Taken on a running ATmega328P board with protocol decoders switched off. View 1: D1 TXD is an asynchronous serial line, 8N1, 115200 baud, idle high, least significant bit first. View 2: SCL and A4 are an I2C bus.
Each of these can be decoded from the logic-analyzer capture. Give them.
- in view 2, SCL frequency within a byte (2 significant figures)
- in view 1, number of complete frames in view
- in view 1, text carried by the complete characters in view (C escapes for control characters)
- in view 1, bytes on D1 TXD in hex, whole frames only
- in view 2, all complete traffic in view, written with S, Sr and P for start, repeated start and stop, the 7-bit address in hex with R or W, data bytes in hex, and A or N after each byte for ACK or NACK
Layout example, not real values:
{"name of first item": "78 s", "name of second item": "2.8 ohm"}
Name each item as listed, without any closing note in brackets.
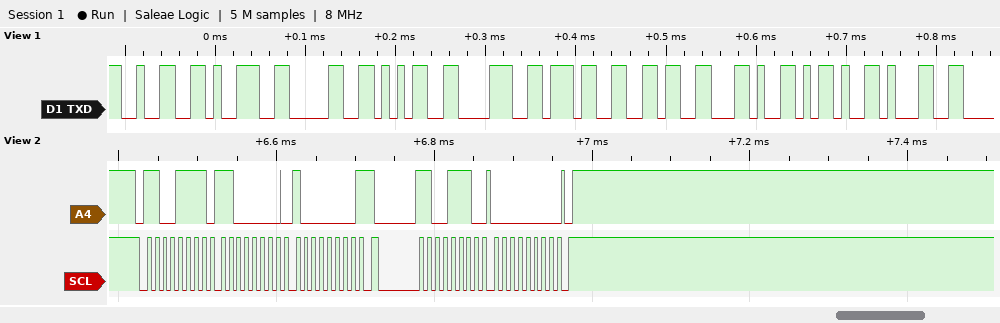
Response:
{"in view 2, SCL frequency within a byte": "100 kHz", "in view 1, number of complete frames in view": "10", "in view 1, text carried by the complete characters in view": "\"2905876,-1\"", "in view 1, bytes on D1 TXD in hex, whole frames only": "32 39 30 35 38 37 36 2C 2D 31", "in view 2, all complete traffic in view, written with S, Sr and P for start, repeated start and stop, the 7-bit address in hex with R or W, data bytes in hex, and A or N after each byte for ACK or NACK": "S 67R A C0 A 80 N Sr 67W A 00 A P"}
